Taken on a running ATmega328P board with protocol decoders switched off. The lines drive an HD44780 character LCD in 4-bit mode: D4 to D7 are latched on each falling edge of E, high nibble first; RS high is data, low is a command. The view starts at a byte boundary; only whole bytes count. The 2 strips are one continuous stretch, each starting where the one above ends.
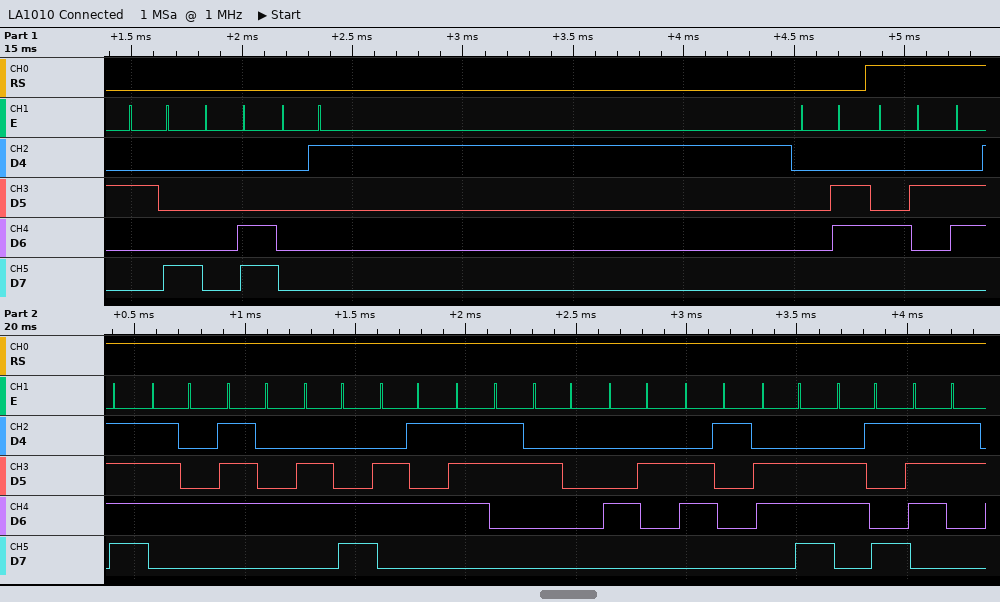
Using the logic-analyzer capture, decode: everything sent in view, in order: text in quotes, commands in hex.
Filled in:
0x28 0x0C 0x01 0x06 "Bottles Banis"
